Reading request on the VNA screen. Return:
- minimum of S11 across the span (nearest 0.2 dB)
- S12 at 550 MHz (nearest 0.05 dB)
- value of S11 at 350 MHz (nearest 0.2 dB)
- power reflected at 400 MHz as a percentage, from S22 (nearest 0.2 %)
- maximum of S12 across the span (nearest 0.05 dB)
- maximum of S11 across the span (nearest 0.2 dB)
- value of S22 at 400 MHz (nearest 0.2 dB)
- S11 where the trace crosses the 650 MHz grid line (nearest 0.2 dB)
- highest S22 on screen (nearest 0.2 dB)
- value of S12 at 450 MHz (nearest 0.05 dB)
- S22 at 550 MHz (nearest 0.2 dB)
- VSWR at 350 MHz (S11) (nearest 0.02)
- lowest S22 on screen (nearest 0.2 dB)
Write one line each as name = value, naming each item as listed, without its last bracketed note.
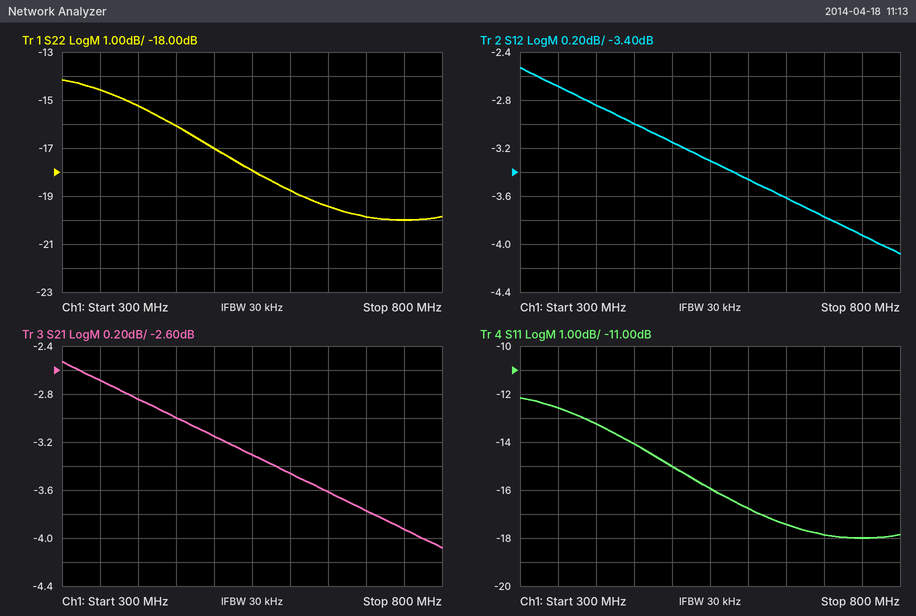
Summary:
minimum of S11 across the span = -18.0 dB
S12 at 550 MHz = -3.30 dB
value of S11 at 350 MHz = -12.6 dB
power reflected at 400 MHz as a percentage, from S22 = 3.0 %
maximum of S12 across the span = -2.55 dB
maximum of S11 across the span = -12.2 dB
value of S22 at 400 MHz = -15.2 dB
S11 where the trace crosses the 650 MHz grid line = -17.4 dB
highest S22 on screen = -14.2 dB
value of S12 at 450 MHz = -3.00 dB
S22 at 550 MHz = -18.0 dB
VSWR at 350 MHz (S11) = 1.62
lowest S22 on screen = -20.0 dB
